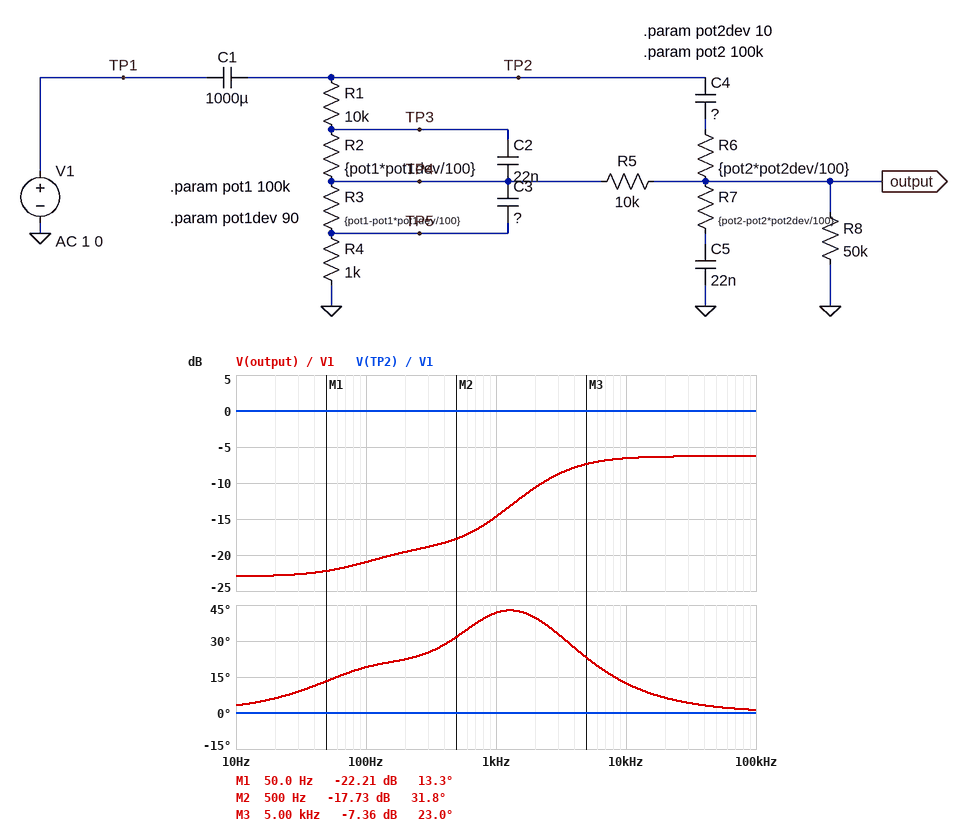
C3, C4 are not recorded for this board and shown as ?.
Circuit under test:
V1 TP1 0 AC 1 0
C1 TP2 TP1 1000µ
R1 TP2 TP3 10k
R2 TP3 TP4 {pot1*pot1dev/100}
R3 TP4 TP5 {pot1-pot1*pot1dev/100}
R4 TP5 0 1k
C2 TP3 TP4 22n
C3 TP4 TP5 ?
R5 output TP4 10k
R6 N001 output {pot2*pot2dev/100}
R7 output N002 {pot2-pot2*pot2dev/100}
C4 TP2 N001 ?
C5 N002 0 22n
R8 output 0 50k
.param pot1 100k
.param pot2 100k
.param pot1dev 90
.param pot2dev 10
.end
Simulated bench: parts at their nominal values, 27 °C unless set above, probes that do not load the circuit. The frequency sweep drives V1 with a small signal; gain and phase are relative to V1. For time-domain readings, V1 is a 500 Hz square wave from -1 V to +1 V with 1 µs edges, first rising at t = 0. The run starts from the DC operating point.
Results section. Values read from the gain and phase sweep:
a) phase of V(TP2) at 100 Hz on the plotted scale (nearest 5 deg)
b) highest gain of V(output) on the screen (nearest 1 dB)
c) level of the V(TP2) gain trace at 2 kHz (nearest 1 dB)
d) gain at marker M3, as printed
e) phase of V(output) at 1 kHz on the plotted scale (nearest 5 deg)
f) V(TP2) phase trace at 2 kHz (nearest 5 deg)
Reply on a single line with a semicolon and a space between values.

0 deg; -6 dB; 0 dB; -7.36 dB; 40 deg; 0 deg
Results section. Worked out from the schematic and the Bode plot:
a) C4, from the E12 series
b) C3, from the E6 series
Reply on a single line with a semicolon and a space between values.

3.3 nF; 150 nF
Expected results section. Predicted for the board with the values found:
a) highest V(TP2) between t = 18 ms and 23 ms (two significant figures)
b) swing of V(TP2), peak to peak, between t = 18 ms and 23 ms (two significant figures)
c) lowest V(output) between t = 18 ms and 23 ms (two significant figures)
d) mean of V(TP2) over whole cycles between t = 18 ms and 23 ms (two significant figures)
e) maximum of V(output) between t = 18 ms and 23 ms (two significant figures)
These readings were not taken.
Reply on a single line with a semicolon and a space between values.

2.0 V; 2.0 V; -800 mV; 1.0 V; 940 mV
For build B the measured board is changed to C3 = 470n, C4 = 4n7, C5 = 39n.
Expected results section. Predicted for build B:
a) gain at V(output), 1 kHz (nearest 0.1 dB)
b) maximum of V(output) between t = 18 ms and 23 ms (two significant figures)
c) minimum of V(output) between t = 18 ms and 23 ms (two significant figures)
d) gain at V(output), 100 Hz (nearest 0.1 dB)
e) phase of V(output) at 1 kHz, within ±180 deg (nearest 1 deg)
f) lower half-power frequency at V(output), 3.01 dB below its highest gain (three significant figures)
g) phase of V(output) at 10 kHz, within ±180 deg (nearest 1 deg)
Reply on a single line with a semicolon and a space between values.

-12.3 dB; 990 mV; -850 mV; -26.1 dB; 50 deg; 1.78 kHz; 9 deg
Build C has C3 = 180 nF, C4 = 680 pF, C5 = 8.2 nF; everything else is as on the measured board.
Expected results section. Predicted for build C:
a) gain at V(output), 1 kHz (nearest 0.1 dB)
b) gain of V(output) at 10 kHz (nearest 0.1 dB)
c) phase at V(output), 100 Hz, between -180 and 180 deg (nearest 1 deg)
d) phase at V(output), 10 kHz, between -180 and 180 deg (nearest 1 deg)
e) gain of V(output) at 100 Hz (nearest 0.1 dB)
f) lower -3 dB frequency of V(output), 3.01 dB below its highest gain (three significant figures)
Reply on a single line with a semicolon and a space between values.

-21.7 dB; -10.4 dB; 6 deg; 42 deg; -22.1 dB; 12.7 kHz
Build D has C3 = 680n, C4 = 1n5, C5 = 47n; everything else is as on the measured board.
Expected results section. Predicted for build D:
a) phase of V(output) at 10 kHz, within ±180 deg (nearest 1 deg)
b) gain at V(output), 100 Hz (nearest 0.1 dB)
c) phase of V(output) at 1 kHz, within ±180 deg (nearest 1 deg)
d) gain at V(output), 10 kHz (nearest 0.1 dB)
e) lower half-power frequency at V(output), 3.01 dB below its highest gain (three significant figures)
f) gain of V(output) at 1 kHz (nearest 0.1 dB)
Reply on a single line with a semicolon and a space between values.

26 deg; -30.1 dB; 53 deg; -7.5 dB; 5.63 kHz; -19.0 dB
